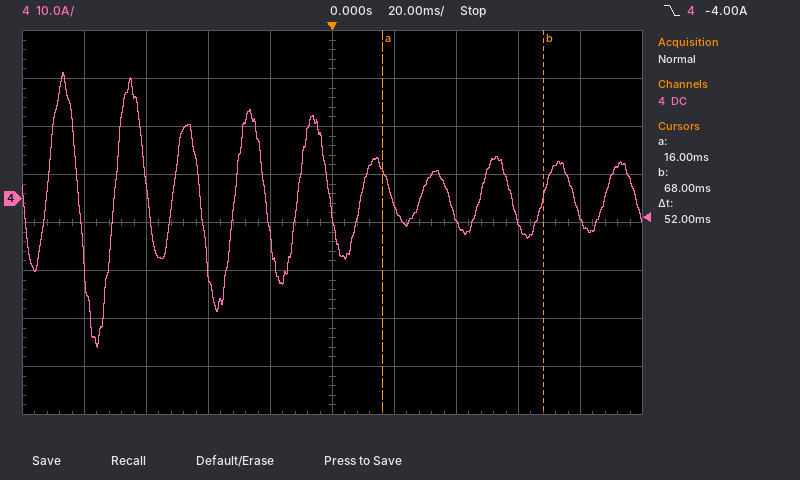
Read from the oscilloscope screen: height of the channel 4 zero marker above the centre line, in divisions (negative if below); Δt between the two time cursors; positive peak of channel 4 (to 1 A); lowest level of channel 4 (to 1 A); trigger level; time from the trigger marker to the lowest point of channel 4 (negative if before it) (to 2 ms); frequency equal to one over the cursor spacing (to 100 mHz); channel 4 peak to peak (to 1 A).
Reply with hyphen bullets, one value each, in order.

- +0.5 div
- 52 ms
- 26 A
- -31 A
- -4.00 A
- -76 ms
- 19.2 Hz
- 57 A
